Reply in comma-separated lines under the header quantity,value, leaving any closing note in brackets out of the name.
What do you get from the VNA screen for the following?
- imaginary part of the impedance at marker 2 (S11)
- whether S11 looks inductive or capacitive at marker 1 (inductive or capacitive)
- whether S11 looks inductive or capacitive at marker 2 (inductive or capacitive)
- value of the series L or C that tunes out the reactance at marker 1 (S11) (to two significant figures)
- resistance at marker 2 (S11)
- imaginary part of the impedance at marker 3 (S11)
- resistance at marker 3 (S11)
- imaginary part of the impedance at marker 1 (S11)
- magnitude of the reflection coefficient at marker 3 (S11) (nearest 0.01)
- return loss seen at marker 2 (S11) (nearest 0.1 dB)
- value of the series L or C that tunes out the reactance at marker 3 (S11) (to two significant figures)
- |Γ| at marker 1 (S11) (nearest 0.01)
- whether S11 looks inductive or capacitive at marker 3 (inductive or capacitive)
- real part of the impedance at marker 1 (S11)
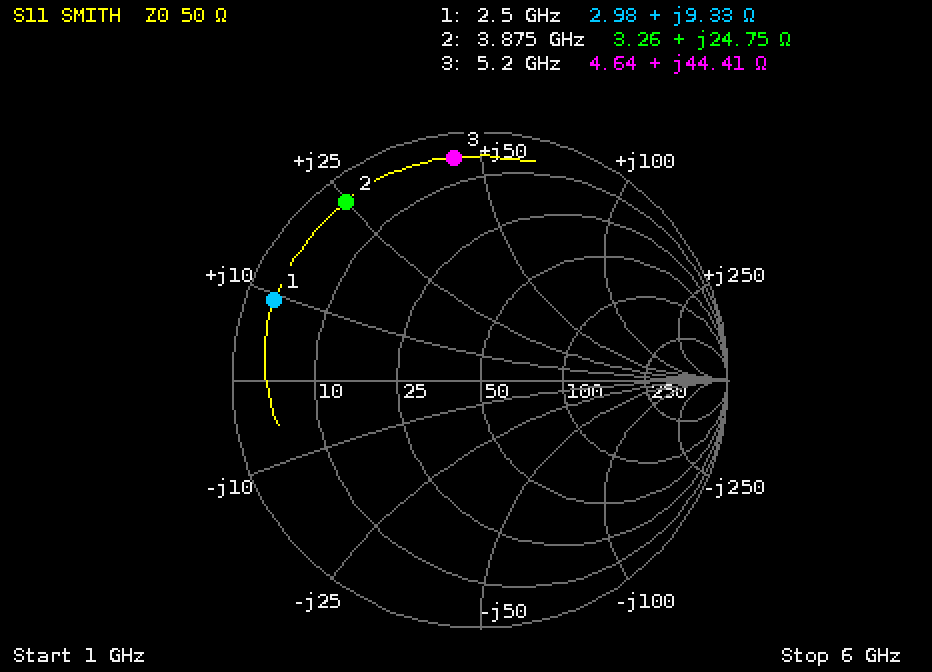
quantity,value
imaginary part of the impedance at marker 2,+24.75 Ω
whether S11 looks inductive or capacitive at marker 1,inductive
whether S11 looks inductive or capacitive at marker 2,inductive
value of the series L or C that tunes out the reactance at marker 1 (S11),6.8 pF
resistance at marker 2,3.26 Ω
imaginary part of the impedance at marker 3,+44.41 Ω
resistance at marker 3,4.64 Ω
imaginary part of the impedance at marker 1,+9.33 Ω
magnitude of the reflection coefficient at marker 3 (S11),0.90
return loss seen at marker 2 (S11),0.9 dB
value of the series L or C that tunes out the reactance at marker 3 (S11),690 fF
|Γ| at marker 1 (S11),0.89
whether S11 looks inductive or capacitive at marker 3,inductive
real part of the impedance at marker 1,2.98 Ω
